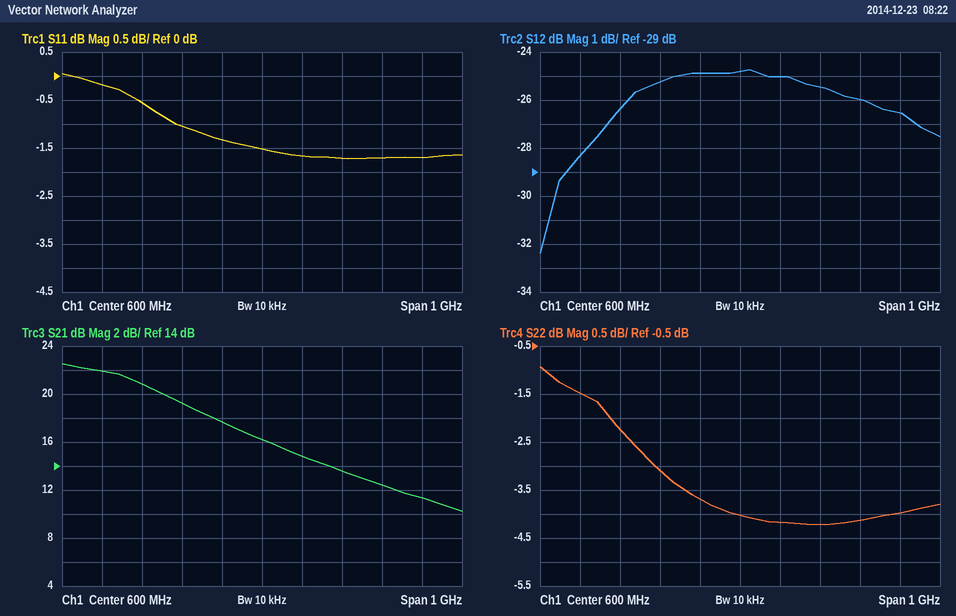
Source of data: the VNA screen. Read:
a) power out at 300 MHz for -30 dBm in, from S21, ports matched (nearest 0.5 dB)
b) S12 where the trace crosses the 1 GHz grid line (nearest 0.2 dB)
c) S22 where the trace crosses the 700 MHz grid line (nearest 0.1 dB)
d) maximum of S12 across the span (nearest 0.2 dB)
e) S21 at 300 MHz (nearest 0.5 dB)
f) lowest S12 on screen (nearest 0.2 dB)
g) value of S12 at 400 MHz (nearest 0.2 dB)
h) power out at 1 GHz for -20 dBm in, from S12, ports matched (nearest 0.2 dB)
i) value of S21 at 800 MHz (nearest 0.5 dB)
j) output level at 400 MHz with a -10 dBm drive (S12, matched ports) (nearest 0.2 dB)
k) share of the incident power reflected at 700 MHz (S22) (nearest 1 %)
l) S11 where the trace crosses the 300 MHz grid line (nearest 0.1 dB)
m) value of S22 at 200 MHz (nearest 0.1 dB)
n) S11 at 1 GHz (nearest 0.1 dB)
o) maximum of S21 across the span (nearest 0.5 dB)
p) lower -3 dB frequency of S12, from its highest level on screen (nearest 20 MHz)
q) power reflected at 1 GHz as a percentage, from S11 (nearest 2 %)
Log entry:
-9.0 dBm
-26.6 dB
-4.2 dB
-24.8 dB
21.0 dB
-32.4 dB
-25.2 dB
-46.6 dBm
13.5 dB
-35.2 dBm
38 %
-0.6 dB
-1.5 dB
-1.7 dB
22.5 dB
240 MHz
68 %
